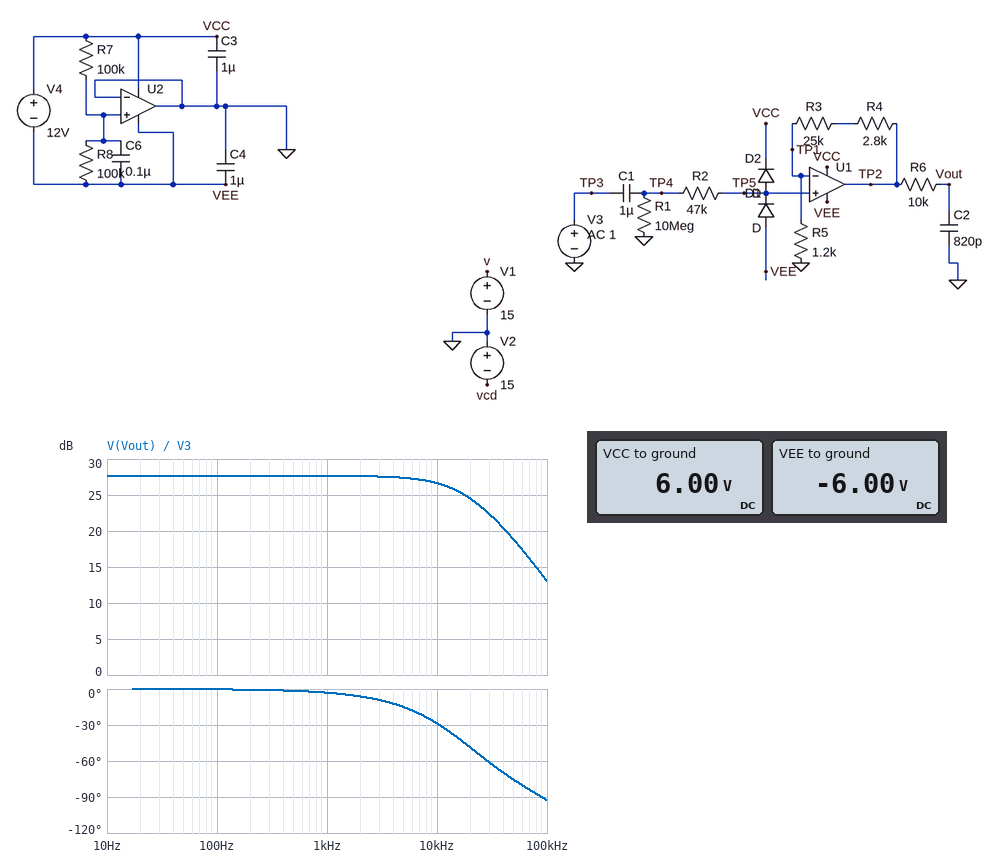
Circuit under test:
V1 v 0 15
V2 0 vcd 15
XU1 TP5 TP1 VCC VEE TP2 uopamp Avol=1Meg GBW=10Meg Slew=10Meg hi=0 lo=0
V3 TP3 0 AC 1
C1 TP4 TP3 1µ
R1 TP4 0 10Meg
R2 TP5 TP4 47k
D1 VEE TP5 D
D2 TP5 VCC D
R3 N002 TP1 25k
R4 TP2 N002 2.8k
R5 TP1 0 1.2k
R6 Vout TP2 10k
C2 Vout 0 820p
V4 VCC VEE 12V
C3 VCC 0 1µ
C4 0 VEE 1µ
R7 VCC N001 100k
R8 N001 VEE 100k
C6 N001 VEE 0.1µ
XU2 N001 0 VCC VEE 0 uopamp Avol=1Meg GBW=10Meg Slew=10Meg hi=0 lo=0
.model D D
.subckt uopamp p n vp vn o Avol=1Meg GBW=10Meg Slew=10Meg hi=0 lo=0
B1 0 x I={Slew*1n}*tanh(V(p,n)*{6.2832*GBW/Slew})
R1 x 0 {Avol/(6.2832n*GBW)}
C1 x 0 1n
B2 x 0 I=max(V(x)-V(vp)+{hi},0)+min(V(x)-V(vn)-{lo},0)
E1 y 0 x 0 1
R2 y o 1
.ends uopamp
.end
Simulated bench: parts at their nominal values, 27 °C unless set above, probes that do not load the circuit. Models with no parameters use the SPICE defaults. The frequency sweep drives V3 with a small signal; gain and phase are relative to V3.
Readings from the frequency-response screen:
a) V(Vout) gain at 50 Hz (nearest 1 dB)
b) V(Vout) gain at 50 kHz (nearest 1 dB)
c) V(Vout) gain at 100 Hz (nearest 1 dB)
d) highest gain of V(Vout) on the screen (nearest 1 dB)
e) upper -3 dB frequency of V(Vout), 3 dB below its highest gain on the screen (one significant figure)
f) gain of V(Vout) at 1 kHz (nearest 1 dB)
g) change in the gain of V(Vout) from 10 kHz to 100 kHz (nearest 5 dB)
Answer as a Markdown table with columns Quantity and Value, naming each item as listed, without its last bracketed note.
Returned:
| Quantity | Value |
|---|---|
| V(Vout) gain at 50 Hz | 28 dB |
| V(Vout) gain at 50 kHz | 19 dB |
| V(Vout) gain at 100 Hz | 28 dB |
| highest gain of V(Vout) on the screen | 28 dB |
| upper -3 dB frequency of V(Vout), 3 dB below its highest gain on the screen | 20 kHz |
| gain of V(Vout) at 1 kHz | 28 dB |
| change in the gain of V(Vout) from 10 kHz to 100 kHz | -15 dB |
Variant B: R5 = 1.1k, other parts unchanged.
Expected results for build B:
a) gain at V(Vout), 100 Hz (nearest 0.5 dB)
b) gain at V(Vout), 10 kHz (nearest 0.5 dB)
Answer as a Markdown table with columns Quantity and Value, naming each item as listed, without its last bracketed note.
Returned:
| Quantity | Value |
|---|---|
| gain at V(Vout), 100 Hz | 28.5 dB |
| gain at V(Vout), 10 kHz | 27.5 dB |
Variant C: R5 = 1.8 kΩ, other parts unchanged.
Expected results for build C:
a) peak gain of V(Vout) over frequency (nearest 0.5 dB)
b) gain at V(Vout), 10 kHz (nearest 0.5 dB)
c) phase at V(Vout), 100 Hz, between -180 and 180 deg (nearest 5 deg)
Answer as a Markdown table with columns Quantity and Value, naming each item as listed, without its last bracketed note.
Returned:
| Quantity | Value |
|---|---|
| peak gain of V(Vout) over frequency | 24.5 dB |
| gain at V(Vout), 10 kHz | 23.5 dB |
| phase at V(Vout), 100 Hz, between -180 and 180 deg | 0 deg |
